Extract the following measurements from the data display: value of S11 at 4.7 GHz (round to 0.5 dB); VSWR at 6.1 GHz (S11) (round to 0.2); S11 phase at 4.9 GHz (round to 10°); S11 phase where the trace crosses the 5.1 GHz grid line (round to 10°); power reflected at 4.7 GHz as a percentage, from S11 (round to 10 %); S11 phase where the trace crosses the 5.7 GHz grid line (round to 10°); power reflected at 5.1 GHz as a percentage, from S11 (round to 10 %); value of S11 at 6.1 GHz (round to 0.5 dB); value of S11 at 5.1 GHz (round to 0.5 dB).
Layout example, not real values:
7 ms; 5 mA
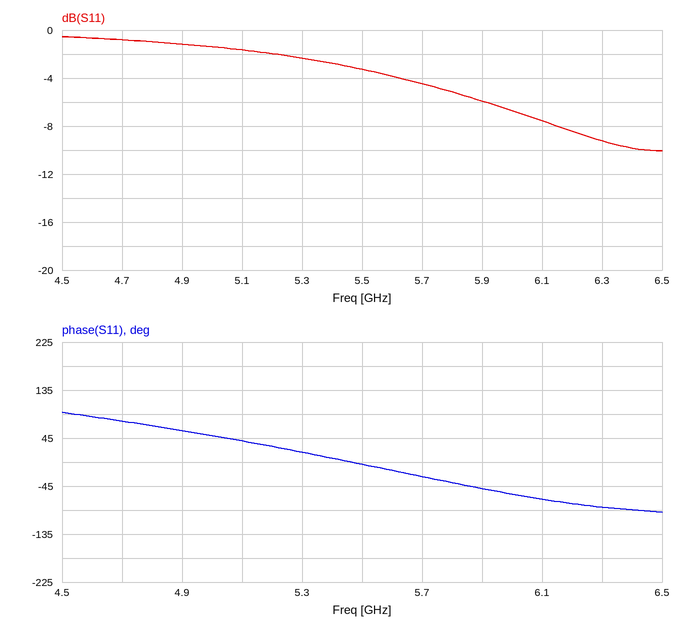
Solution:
-1.0 dB; 2.4; 60°; 40°; 80 %; -30°; 70 %; -7.5 dB; -1.5 dB
